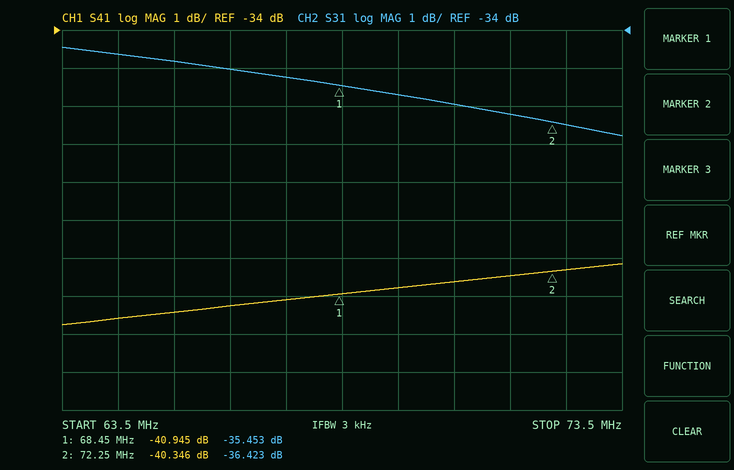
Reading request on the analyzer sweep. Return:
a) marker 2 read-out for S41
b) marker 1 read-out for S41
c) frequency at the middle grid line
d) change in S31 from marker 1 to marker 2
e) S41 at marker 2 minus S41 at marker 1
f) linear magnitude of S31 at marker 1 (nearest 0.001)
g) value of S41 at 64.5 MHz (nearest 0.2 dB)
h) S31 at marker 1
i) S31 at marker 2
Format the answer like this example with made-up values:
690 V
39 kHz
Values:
-40.346 dB
-40.945 dB
68.5 MHz
-0.970 dB
0.599 dB
0.017
-41.6 dB
-35.453 dB
-36.423 dB
